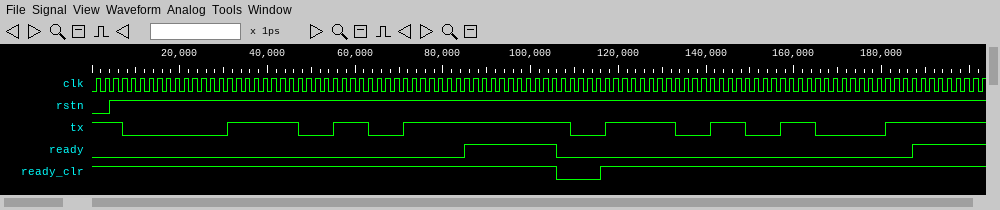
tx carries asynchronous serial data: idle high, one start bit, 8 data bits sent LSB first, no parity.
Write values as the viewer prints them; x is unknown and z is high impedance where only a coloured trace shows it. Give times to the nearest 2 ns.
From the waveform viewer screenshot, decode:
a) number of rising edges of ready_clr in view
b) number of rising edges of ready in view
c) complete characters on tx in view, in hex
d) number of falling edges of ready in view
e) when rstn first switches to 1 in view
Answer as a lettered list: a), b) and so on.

a) 1
b) 2
c) AC, 2B
d) 1
e) 4 ns
